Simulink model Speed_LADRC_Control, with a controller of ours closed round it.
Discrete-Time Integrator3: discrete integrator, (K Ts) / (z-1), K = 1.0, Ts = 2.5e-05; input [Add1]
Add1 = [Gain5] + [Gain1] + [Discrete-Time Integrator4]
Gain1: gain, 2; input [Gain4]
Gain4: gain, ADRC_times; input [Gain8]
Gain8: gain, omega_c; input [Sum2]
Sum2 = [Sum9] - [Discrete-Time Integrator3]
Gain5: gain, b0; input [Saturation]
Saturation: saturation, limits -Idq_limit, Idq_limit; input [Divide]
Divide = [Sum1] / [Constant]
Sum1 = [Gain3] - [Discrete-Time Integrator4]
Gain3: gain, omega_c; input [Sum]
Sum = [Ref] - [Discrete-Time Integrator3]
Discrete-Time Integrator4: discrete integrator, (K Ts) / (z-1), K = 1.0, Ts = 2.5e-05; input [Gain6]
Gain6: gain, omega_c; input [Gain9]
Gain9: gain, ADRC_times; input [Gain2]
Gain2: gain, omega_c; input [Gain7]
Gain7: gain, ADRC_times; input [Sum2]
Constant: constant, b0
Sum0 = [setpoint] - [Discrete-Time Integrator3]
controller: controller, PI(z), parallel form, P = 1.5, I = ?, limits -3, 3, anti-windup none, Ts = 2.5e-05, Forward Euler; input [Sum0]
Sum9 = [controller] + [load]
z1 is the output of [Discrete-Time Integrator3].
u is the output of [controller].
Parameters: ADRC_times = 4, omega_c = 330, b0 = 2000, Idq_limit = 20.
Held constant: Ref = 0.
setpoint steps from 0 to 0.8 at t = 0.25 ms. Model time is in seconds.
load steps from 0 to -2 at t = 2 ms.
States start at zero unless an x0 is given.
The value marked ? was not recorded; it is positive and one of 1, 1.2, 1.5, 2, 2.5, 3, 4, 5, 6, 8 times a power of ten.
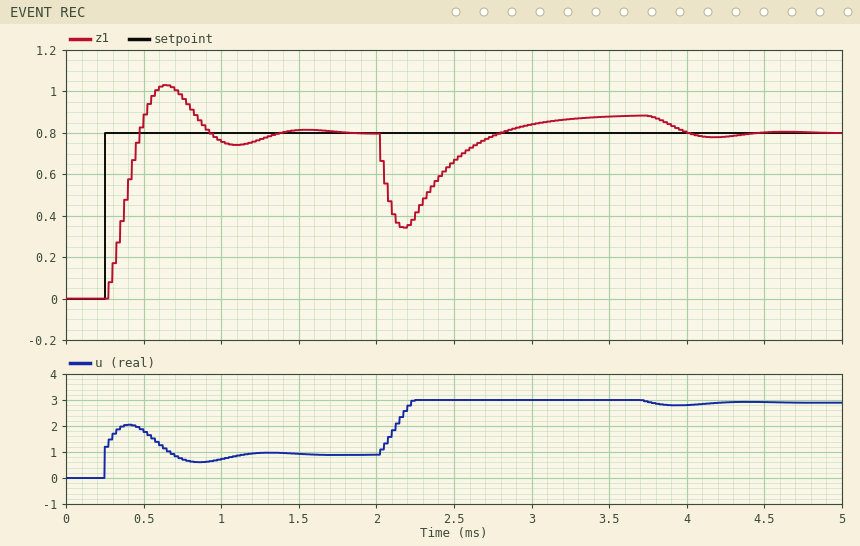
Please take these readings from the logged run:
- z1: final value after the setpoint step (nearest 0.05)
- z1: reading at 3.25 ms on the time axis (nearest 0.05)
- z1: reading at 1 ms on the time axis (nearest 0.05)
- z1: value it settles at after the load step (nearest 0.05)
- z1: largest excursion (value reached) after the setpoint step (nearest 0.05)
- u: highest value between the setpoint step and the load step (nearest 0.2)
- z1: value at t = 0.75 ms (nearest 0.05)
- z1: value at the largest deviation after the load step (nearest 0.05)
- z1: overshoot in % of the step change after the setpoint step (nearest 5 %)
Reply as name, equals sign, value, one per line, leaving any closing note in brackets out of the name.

z1: final value after the setpoint step = 0.80
z1: reading at 3.25 ms on the time axis = 0.85
z1: reading at 1 ms on the time axis = 0.75
z1: value it settles at after the load step = 0.80
z1: largest excursion (value reached) after the setpoint step = 1.05
u: highest value between the setpoint step and the load step = 2.0
z1: value at t = 0.75 ms = 0.95
z1: value at the largest deviation after the load step = 0.35
z1: overshoot in % of the step change after the setpoint step = 30 %
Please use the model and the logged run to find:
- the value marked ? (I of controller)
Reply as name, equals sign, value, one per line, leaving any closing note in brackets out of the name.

the value marked ? = 20000
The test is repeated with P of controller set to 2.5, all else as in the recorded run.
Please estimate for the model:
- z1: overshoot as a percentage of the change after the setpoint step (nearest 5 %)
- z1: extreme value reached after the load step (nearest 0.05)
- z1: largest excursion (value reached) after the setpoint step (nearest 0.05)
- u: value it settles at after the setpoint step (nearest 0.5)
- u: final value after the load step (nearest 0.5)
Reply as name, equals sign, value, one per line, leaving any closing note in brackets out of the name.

z1: overshoot as a percentage of the change after the setpoint step = 15 %
z1: extreme value reached after the load step = 0.40
z1: largest excursion (value reached) after the setpoint step = 0.95
u: value it settles at after the setpoint step = 1.0
u: final value after the load step = 3.0
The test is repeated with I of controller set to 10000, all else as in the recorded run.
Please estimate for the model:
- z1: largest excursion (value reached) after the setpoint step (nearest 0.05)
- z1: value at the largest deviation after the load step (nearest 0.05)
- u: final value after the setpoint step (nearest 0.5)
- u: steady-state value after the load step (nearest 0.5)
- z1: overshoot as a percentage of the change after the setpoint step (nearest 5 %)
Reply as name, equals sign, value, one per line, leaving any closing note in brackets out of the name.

z1: largest excursion (value reached) after the setpoint step = 0.90
z1: value at the largest deviation after the load step = 0.30
u: final value after the setpoint step = 1.0
u: steady-state value after the load step = 3.0
z1: overshoot as a percentage of the change after the setpoint step = 10 %
